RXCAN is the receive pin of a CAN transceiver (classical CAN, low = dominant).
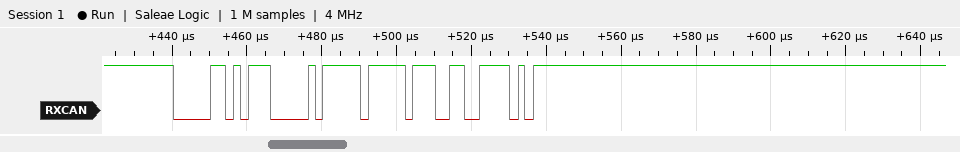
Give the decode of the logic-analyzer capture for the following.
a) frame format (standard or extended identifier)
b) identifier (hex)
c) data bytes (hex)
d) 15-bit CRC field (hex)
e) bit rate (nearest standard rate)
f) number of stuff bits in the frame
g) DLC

standard
0x057
FF
0x799E
500 kbit/s
4
1
